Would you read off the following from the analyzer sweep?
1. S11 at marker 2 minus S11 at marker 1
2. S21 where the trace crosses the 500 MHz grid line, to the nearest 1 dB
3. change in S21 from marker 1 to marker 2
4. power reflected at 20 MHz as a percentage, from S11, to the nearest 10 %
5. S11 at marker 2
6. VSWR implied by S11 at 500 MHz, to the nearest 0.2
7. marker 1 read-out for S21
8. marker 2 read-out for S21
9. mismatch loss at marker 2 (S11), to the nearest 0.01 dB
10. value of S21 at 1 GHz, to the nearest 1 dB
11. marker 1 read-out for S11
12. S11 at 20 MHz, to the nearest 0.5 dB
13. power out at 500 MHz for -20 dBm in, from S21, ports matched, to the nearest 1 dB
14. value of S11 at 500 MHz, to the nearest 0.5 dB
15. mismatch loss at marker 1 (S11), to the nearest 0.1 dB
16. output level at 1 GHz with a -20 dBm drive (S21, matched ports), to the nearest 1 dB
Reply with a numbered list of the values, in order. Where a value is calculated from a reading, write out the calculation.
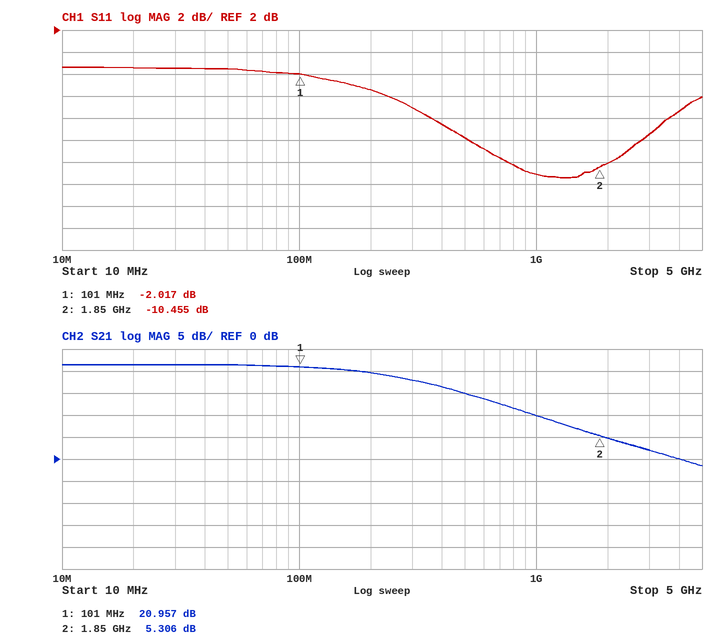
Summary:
1. -10.455 − (-2.017) = -8.438 dB
2. 15 dB
3. 5.306 − (20.957) = -15.651 dB
4. 10^(-1.5/10) ≈ 70.8 %, so 70 % to the nearest 10 %
5. -10.455 dB
6. |Γ| = 10^(-8/20) = 0.3981; VSWR = (1 + 0.3981)/(1 − 0.3981) ≈ 2.32, so 2.4 to the nearest 0.2
7. 20.957 dB
8. 5.306 dB
9. −10 log10(1 − 10^(-10.455/10)) ≈ 0.41 dB
10. 10 dB
11. -2.017 dB
12. -1.5 dB
13. -20 dBm + (15 dB) = -5 dBm
14. -8.0 dB
15. −10 log10(1 − 10^(-2.017/10)) ≈ 4.3 dB
16. -20 dBm + (10 dB) = -10 dBm
